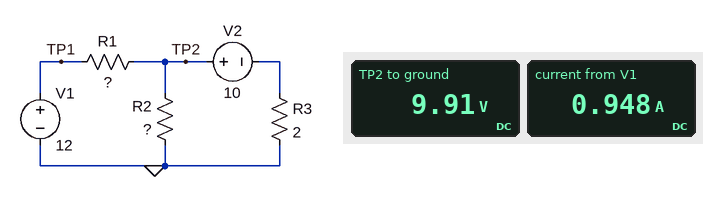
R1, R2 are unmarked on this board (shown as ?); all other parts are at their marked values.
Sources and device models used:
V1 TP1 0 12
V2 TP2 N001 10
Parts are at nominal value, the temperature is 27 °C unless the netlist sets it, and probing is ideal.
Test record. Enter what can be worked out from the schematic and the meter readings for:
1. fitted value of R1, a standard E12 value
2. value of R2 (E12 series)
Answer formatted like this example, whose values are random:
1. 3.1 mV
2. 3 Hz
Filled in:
1. 2.2 Ω
2. 10 Ω
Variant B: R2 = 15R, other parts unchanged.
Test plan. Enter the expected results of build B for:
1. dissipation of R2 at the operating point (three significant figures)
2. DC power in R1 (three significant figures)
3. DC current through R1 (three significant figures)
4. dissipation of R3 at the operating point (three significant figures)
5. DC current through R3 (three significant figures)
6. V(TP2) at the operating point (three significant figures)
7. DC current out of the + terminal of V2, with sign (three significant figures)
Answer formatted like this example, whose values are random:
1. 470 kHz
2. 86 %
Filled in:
1. 6.99 W
2. 1.41 W
3. 801 mA
4. 28.2 mW
5. 119 mA
6. 10.2 V
7. -119 mA
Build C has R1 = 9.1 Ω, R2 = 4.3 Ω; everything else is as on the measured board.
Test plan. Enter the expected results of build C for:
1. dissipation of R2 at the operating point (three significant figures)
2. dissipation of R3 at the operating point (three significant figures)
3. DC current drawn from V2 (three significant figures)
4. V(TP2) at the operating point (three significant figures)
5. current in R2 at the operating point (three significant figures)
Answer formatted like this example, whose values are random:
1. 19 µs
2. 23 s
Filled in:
1. 13.1 W
2. 3.12 W
3. 1.25 A
4. 7.50 V
5. 1.74 A
